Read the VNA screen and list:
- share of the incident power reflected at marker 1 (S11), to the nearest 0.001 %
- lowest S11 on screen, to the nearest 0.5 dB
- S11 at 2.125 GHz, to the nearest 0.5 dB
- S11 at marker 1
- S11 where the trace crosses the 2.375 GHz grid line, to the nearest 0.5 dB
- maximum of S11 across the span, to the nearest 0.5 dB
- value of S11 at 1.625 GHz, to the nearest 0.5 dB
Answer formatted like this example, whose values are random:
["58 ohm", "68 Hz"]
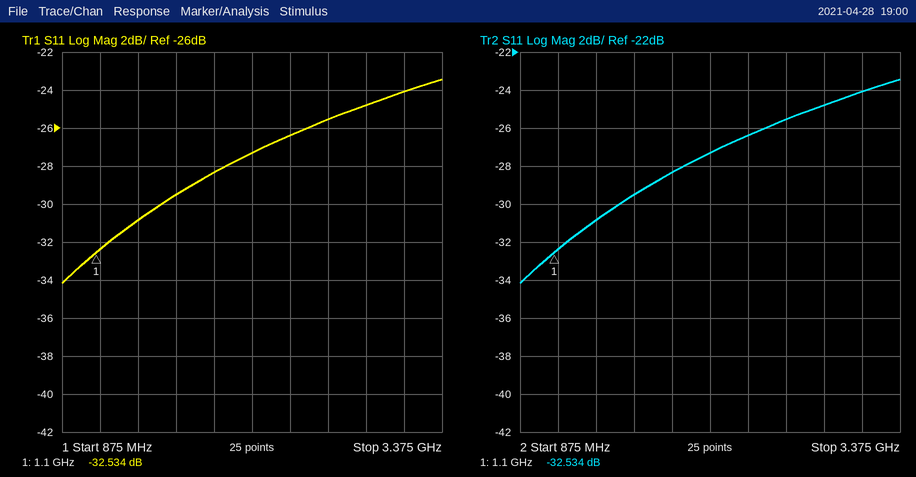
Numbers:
["0.056 %", "-34.0 dB", "-27.5 dB", "-32.534 dB", "-26.5 dB", "-23.5 dB", "-29.5 dB"]
